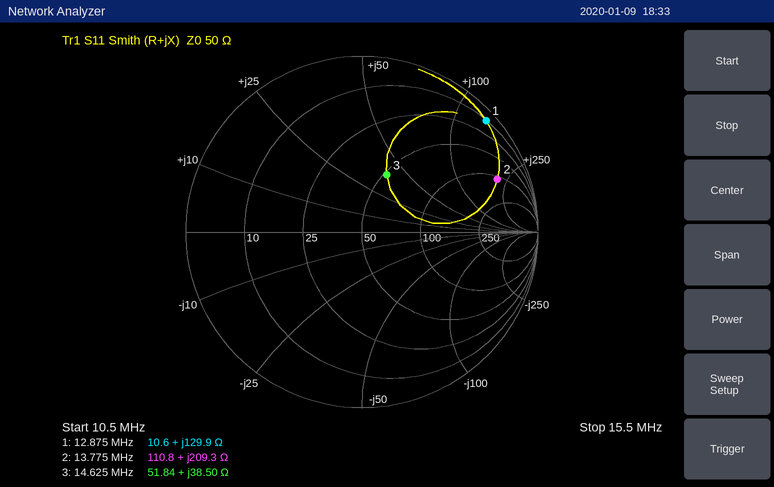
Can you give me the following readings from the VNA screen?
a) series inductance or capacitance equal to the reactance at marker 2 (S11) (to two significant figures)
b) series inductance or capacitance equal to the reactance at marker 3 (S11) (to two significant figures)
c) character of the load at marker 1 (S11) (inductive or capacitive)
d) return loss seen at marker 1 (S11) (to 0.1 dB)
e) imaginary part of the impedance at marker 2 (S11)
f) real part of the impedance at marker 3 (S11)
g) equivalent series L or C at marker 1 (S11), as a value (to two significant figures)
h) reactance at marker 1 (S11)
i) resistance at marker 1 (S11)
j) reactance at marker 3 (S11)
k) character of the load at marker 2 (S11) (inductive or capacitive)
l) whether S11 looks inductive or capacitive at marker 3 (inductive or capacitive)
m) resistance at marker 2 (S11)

2.4 µH
420 nH
inductive
0.5 dB
+209.3 Ω
51.84 Ω
1.6 µH
+129.9 Ω
10.6 Ω
+38.50 Ω
inductive
inductive
110.8 Ω
